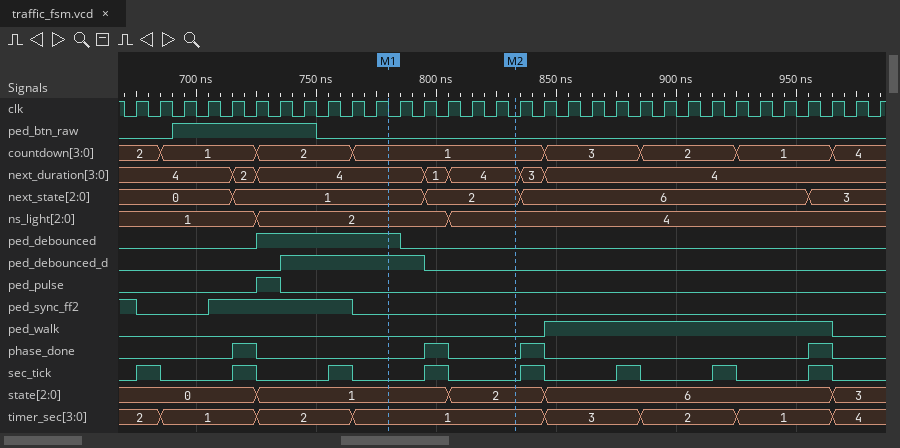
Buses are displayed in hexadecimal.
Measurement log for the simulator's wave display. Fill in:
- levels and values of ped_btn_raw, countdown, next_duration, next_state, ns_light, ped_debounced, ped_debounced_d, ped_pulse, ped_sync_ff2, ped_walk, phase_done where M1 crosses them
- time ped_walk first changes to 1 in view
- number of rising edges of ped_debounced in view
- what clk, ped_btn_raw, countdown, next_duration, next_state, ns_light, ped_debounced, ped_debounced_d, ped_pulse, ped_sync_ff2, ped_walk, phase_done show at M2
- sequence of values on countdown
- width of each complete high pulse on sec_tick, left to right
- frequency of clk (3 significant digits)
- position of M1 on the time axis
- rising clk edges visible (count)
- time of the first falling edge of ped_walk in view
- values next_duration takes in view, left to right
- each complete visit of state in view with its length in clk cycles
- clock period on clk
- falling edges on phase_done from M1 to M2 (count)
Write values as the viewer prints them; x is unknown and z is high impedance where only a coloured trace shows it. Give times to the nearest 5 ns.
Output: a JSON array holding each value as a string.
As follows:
["ped_btn_raw=0, countdown=1, next_duration=4, next_state=1, ns_light=2, ped_debounced=1, ped_debounced_d=1, ped_pulse=0, ped_sync_ff2=0, ped_walk=0, phase_done=0", "845 ns", "1", "clk=0, ped_btn_raw=0, countdown=1, next_duration=4, next_state=2, ns_light=4, ped_debounced=0, ped_debounced_d=0, ped_pulse=0, ped_sync_ff2=0, ped_walk=0, phase_done=0", "2, 1, 2, 1, 3, 2, 1, 4", "10 ns, 10 ns, 10 ns, 10 ns, 10 ns, 10 ns, 10 ns, 10 ns", "100 MHz", "780 ns", "32", "965 ns", "4, 2, 4, 1, 4, 3, 4", "1: 8, 2: 4, 6: 12", "10 ns", "1"]
